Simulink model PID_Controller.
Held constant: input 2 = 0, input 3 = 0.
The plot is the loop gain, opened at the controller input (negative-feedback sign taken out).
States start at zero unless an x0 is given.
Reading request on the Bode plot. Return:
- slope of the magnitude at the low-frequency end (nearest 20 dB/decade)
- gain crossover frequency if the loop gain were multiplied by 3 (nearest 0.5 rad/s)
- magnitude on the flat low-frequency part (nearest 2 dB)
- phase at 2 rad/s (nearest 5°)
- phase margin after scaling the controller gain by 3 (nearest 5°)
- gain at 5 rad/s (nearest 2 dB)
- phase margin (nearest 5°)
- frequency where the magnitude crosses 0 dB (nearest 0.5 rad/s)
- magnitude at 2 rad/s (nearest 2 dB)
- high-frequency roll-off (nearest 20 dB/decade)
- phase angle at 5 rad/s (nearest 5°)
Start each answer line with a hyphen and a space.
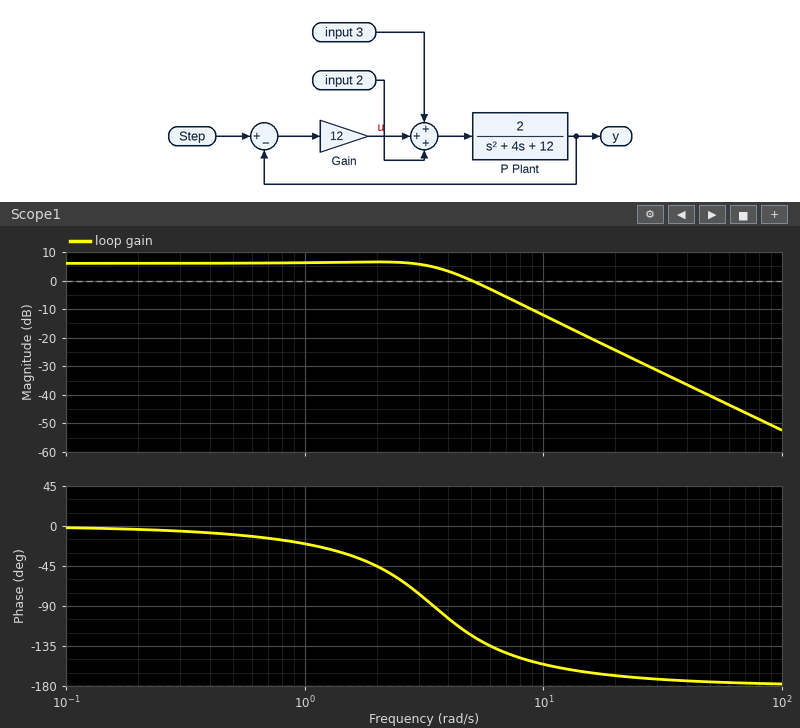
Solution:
- 0 dB/decade
- 8.5 rad/s
- 6 dB
- -45°
- 30°
- 0 dB
- 55°
- 5.0 rad/s
- 6 dB
- -40 dB/decade
- -125°
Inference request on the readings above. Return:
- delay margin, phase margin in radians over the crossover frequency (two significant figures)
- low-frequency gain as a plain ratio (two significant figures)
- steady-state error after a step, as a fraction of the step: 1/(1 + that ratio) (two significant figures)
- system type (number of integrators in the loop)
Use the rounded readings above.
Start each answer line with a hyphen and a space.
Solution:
- 0.19 s
- 2.0
- 0.33
- 0
